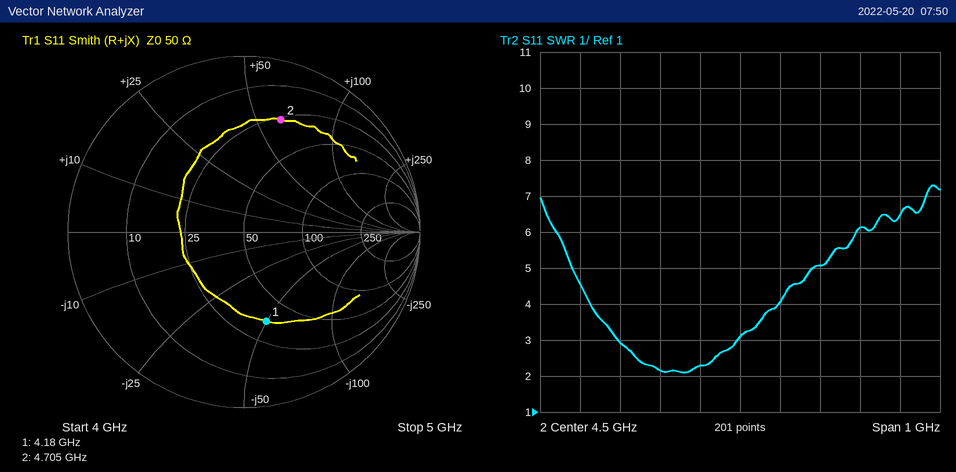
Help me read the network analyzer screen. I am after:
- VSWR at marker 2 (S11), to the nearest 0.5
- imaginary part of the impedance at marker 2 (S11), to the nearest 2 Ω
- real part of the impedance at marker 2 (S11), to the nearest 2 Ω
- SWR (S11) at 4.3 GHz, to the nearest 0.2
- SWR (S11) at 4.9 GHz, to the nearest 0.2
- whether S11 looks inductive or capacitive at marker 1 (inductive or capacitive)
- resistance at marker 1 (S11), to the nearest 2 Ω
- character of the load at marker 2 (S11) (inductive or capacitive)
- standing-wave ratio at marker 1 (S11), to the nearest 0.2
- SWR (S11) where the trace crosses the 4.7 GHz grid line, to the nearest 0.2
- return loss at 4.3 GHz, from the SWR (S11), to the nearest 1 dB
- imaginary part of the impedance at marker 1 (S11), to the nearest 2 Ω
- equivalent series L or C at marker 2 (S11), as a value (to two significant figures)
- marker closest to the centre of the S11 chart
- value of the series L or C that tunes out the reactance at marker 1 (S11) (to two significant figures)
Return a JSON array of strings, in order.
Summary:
["5.0", "+62 Ω", "26 Ω", "2.2", "6.4", "capacitive", "36 Ω", "inductive", "3.2", "5.0", "9 dB", "-50 Ω", "2.1 nH", "marker 1", "1.9 nH"]
